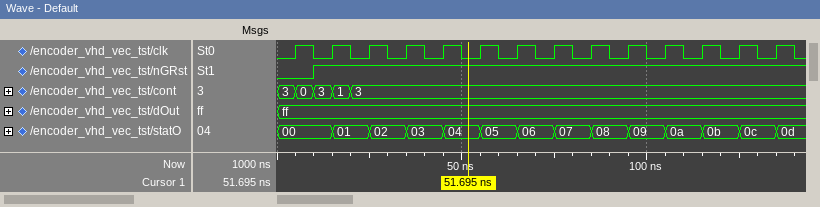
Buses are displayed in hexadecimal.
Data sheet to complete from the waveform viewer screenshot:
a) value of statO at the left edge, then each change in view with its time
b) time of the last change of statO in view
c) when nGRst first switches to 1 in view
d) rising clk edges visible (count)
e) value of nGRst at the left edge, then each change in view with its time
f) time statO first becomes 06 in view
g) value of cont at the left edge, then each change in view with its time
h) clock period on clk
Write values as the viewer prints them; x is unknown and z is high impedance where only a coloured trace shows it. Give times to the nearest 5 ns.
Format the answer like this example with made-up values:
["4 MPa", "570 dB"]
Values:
["00, 01 at 15 ns, 02 at 25 ns, 03 at 35 ns, 04 at 45 ns, 05 at 55 ns, 06 at 65 ns, 07 at 75 ns, 08 at 85 ns, 09 at 95 ns, 0a at 105 ns, 0b at 115 ns, 0c at 125 ns, 0d at 135 ns", "135 ns", "10 ns", "14", "0, 1 at 10 ns", "65 ns", "3, 0 at 5 ns, 3 at 10 ns, 1 at 15 ns, 3 at 20 ns", "10 ns"]
